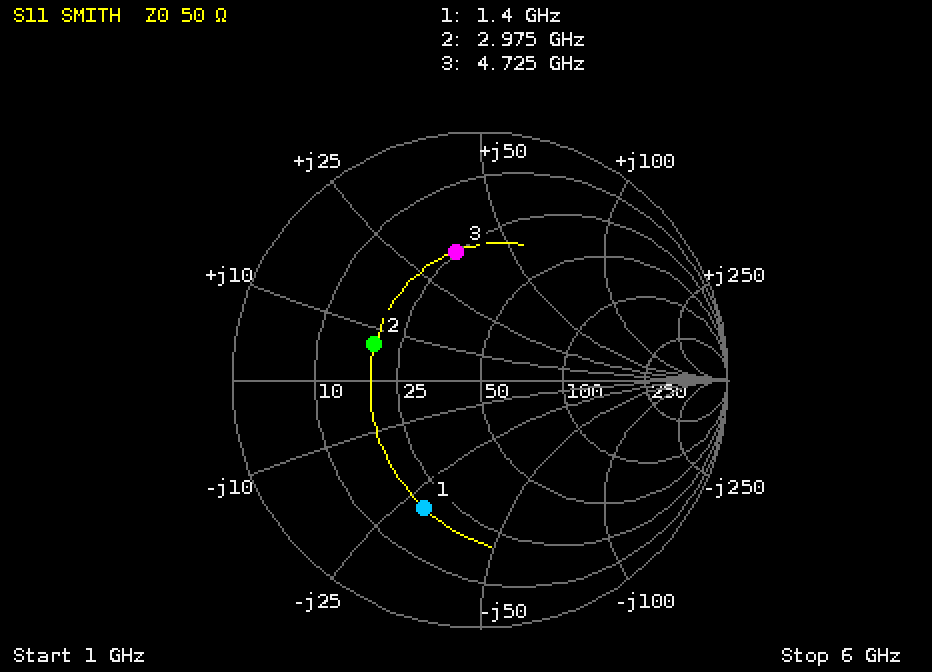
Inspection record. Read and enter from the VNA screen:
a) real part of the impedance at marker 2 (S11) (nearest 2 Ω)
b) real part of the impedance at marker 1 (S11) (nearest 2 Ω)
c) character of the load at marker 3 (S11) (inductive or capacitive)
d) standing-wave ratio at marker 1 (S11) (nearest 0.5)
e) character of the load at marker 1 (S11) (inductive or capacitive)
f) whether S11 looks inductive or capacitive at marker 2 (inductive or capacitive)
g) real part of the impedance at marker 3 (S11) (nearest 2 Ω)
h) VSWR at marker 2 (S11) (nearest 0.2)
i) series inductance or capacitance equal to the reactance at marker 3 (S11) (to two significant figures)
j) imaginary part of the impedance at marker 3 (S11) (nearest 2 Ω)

20 Ω
20 Ω
inductive
3.5
capacitive
inductive
24 Ω
2.6
1.2 nH
+36 Ω
